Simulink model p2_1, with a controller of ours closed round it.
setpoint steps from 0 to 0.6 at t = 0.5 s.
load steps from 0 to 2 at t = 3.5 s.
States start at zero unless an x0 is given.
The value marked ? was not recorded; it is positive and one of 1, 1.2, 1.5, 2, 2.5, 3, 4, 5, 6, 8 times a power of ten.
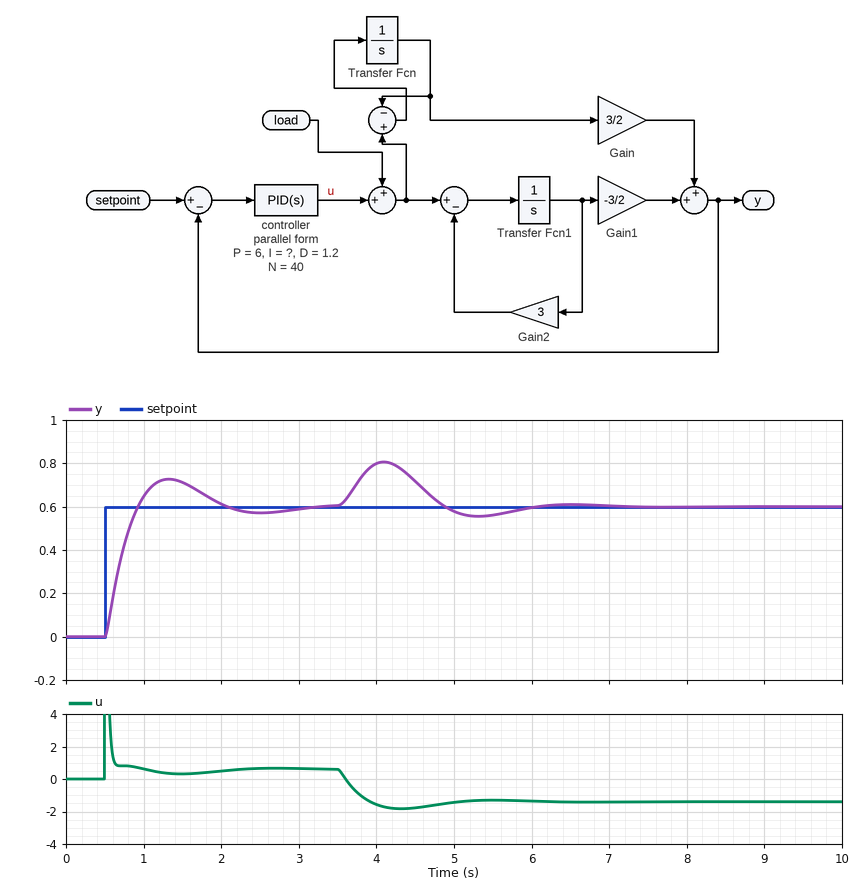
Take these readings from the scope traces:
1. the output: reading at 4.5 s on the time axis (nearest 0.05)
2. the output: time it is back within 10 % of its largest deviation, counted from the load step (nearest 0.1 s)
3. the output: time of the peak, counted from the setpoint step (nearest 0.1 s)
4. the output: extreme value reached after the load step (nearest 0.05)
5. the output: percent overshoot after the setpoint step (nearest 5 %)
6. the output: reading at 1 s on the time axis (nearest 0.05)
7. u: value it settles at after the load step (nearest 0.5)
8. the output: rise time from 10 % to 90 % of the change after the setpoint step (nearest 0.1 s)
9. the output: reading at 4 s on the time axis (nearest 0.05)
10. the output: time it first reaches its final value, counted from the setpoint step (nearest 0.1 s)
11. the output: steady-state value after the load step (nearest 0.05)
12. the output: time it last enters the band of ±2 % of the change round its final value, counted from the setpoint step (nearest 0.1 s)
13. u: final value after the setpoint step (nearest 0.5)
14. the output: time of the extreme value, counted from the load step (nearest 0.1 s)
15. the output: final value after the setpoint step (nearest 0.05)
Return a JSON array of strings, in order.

["0.70", "2.3 s", "0.8 s", "0.80", "20 %", "0.65", "-1.5", "0.3 s", "0.80", "0.4 s", "0.60", "2.5 s", "0.5", "0.6 s", "0.60"]
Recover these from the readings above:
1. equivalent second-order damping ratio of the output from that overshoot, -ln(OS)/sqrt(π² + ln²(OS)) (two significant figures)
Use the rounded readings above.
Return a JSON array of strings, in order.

["0.46"]
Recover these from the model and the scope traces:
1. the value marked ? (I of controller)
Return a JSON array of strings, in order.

["15"]
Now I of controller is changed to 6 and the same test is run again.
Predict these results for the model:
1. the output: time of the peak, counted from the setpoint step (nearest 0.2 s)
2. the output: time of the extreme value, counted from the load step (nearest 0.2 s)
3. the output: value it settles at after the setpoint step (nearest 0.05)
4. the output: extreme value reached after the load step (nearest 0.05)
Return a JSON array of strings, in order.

["1.0 s", "0.8 s", "0.60", "0.85"]
